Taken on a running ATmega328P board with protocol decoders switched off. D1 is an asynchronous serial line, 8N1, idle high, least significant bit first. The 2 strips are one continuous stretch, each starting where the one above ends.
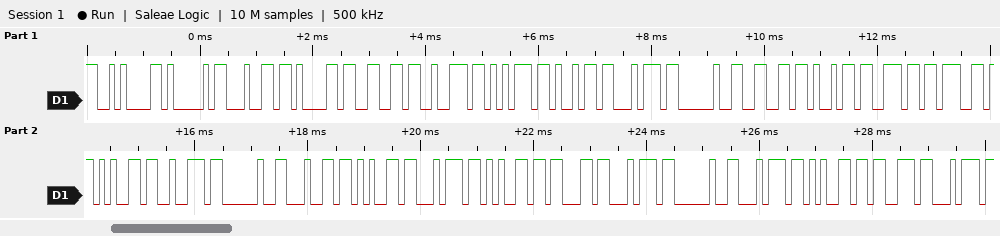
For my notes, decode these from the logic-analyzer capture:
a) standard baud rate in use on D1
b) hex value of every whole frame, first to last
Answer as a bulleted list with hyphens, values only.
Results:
- 9600 baud
- 0A 41 64 61 66 72 75 69 74 20 66 69 6E 67 65 72 20 64 65 74 65 63 74 20 74 65 73 74
